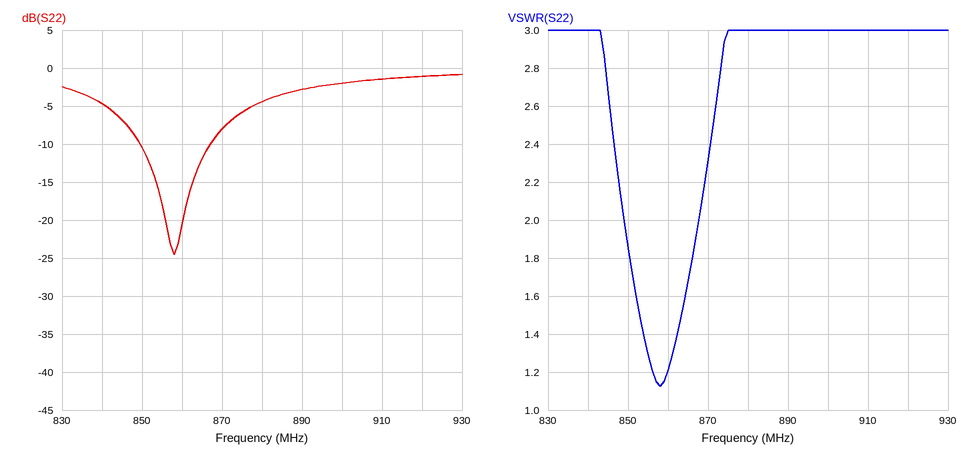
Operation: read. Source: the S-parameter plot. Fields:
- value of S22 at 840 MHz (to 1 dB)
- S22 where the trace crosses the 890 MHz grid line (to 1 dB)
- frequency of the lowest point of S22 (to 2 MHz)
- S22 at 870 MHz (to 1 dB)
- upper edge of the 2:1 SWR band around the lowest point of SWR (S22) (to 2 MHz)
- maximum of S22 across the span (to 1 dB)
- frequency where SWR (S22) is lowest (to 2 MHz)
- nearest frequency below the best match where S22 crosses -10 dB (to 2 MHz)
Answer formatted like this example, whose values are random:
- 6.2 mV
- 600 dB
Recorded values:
- -5 dB
- -3 dB
- 858 MHz
- -8 dB
- 868 MHz
- -1 dB
- 858 MHz
- 850 MHz
